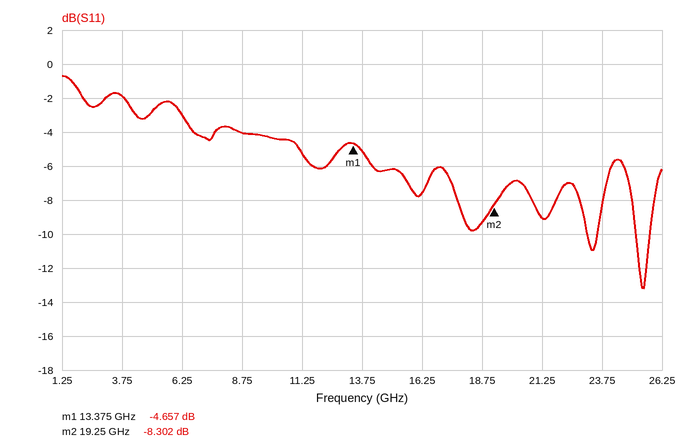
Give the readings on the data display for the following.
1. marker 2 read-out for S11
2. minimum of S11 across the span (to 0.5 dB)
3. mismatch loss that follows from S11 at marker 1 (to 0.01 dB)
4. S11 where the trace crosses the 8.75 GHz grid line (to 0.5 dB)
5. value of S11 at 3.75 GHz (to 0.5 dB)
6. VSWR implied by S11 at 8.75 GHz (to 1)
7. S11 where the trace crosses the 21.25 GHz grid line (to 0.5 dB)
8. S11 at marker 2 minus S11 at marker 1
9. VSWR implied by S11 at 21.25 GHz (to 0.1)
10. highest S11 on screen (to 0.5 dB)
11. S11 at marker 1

-8.302 dB
-13.0 dB
1.82 dB
-4.0 dB
-2.0 dB
4
-9.0 dB
-3.645 dB
2.1
-0.5 dB
-4.657 dB
